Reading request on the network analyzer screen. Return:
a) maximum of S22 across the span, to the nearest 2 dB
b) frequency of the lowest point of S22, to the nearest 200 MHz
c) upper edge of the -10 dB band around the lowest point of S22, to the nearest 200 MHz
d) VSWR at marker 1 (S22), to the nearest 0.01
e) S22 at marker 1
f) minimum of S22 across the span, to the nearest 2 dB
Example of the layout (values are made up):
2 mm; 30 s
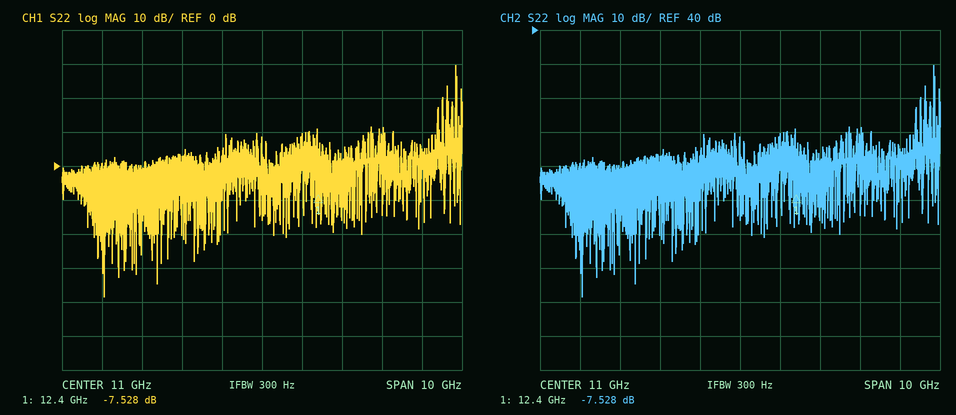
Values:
30 dB; 7.0 GHz; 7.0 GHz; 2.45; -7.528 dB; -38 dB
